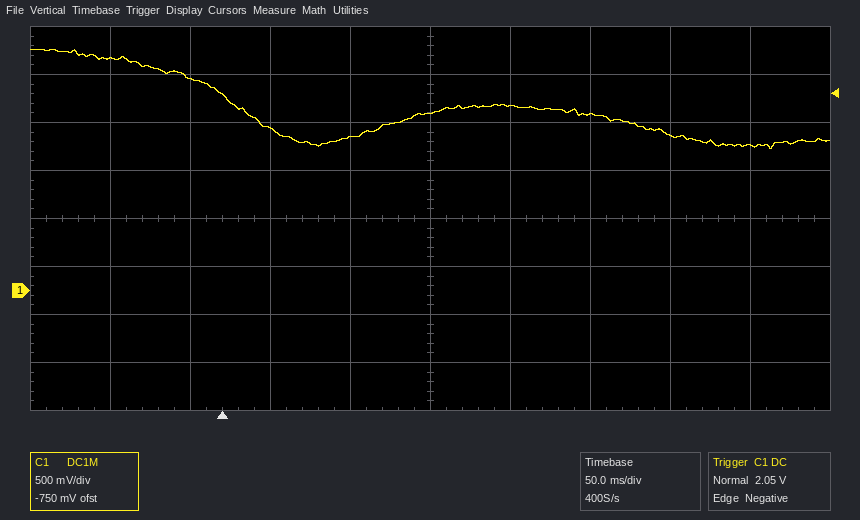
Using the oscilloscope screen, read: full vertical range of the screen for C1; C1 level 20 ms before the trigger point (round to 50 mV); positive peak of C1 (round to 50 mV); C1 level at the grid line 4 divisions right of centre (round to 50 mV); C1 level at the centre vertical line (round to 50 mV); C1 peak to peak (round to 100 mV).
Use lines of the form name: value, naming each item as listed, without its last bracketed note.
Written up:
full vertical range of the screen for C1: 4 V
C1 level 20 ms before the trigger point: 2.20 V
positive peak of C1: 2.50 V
C1 level at the grid line 4 divisions right of centre: 1.50 V
C1 level at the centre vertical line: 1.85 V
C1 peak to peak: 1.00 V
